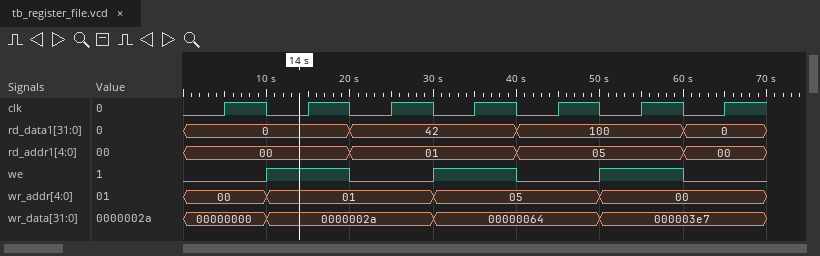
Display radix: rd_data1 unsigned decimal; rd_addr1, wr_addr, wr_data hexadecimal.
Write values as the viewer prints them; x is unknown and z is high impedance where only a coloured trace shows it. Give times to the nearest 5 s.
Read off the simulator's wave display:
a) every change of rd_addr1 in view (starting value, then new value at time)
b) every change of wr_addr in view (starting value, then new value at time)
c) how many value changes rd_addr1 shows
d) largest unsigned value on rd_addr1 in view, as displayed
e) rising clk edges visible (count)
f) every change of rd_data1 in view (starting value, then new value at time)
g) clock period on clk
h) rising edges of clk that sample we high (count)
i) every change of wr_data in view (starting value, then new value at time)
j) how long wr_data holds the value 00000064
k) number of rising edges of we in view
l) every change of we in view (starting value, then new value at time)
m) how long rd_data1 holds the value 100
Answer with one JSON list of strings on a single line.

["00, 01 at 20 s, 05 at 40 s, 00 at 60 s", "00, 01 at 10 s, 05 at 30 s, 00 at 50 s", "3", "05", "7", "0, 42 at 20 s, 100 at 40 s, 0 at 60 s", "10 s", "3", "00000000, 0000002a at 10 s, 00000064 at 30 s, 000003e7 at 50 s", "20 s", "3", "0, 1 at 10 s, 0 at 20 s, 1 at 30 s, 0 at 40 s, 1 at 50 s, 0 at 60 s", "20 s"]
